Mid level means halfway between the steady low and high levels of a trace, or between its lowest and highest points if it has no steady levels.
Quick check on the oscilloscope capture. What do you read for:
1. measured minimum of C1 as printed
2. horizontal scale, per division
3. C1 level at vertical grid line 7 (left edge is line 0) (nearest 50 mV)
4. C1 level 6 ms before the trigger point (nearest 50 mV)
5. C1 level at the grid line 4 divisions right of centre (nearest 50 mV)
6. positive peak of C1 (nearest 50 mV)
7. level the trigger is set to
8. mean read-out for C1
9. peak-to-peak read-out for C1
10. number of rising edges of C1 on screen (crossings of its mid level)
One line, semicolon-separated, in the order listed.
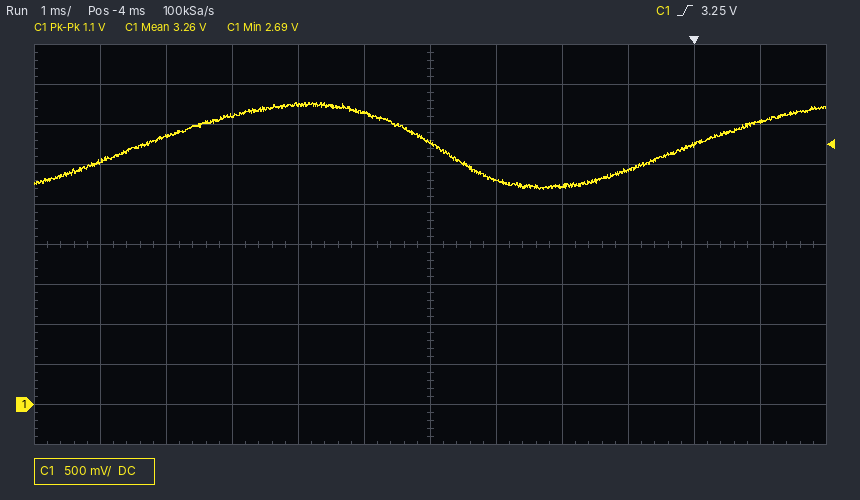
2.69 V; 1 ms; 2.80 V; 3.75 V; 3.25 V; 3.80 V; 3.25 V; 3.26 V; 1.1 V; 2
